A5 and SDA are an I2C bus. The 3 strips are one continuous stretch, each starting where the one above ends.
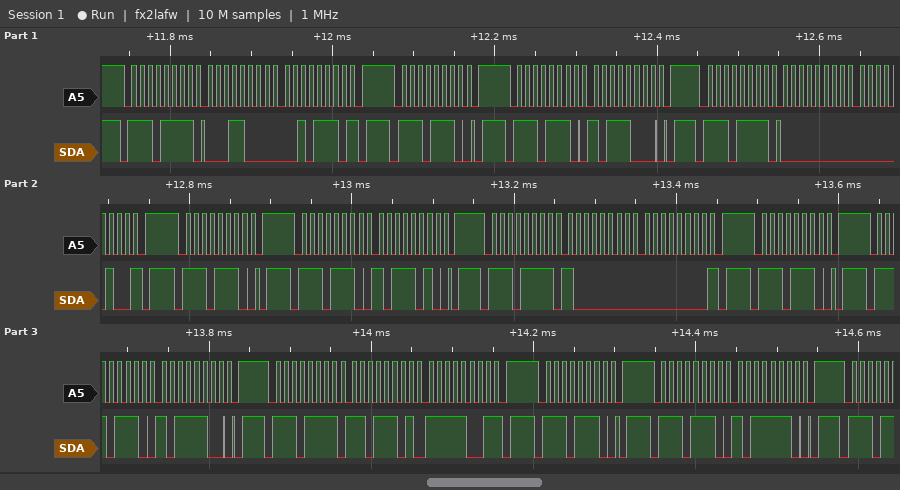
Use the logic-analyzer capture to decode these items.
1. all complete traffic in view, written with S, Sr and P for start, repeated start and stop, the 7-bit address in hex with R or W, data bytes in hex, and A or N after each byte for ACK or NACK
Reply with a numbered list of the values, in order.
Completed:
1. S 77R A 18 A 2E N P S 77W A P S 77W A B8 A P S 77R A 00 A 04 N P S 77W A P S 77W A BA A P S 77R A 80 A 00 N P S 77W A P S 77W A BC A P S 77R A DD A F9 N P S 77W A P S 77W A BE A P
